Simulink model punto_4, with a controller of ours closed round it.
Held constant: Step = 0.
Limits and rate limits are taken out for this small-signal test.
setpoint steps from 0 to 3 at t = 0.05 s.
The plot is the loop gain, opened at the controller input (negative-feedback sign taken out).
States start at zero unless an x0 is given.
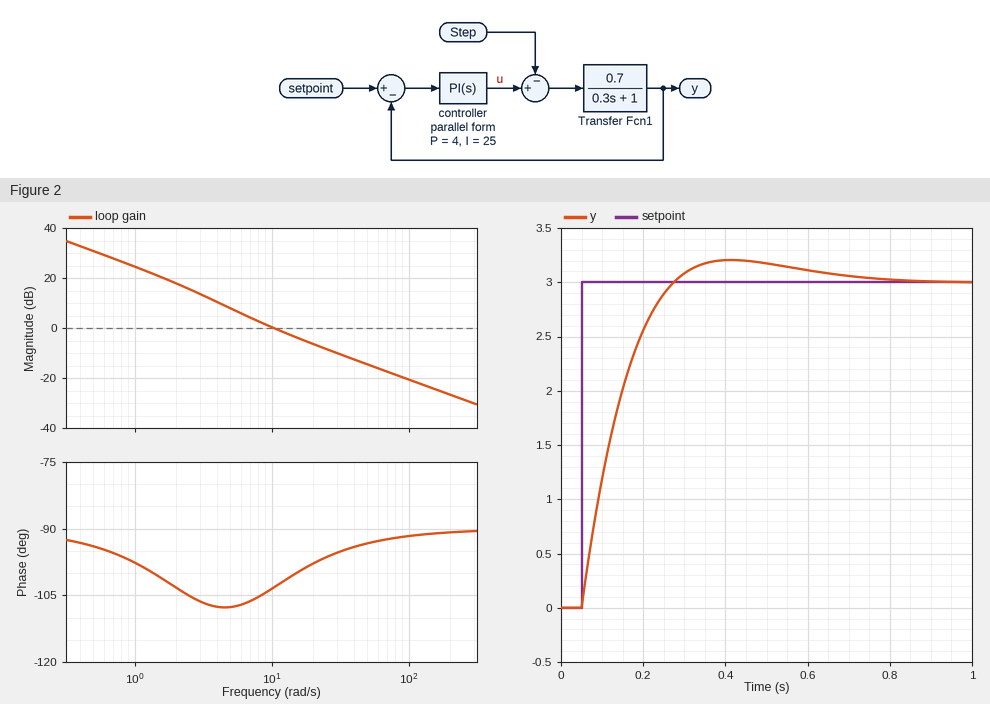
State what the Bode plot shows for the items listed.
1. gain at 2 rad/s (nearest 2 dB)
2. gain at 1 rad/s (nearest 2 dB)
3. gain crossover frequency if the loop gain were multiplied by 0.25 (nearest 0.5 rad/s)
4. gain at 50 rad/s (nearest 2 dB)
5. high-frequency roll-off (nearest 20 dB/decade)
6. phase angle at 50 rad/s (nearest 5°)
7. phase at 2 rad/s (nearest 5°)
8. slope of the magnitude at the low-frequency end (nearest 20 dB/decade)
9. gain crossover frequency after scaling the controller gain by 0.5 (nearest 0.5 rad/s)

18 dB
24 dB
3.5 rad/s
-14 dB
-20 dB/decade
-95°
-105°
-20 dB/decade
6.0 rad/s
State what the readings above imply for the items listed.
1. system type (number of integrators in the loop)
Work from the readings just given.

1
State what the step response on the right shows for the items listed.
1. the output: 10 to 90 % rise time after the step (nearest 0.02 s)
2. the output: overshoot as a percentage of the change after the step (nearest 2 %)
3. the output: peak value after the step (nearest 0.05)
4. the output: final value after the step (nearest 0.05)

0.16 s
6 %
3.20
3.00
